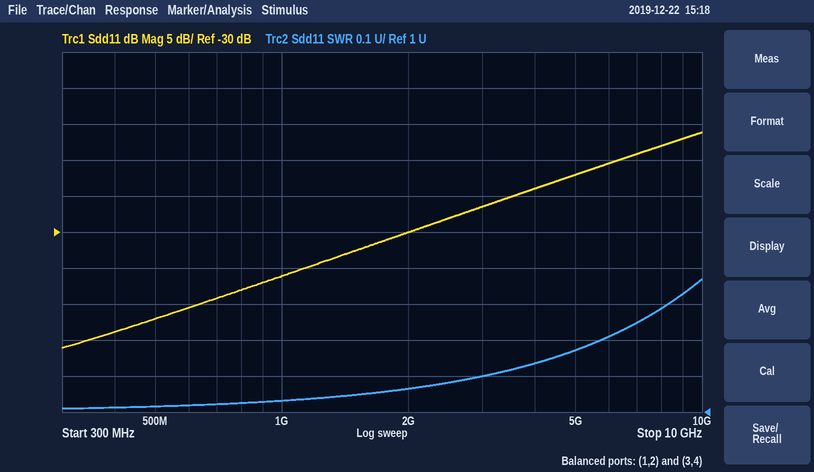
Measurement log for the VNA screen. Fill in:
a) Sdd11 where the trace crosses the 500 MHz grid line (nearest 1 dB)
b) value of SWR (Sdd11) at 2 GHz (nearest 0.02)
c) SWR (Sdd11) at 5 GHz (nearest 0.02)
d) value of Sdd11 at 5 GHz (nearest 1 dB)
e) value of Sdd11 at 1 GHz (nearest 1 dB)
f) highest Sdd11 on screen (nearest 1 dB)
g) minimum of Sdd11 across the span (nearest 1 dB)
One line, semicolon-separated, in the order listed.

-42 dB; 1.06; 1.18; -22 dB; -36 dB; -16 dB; -46 dB
